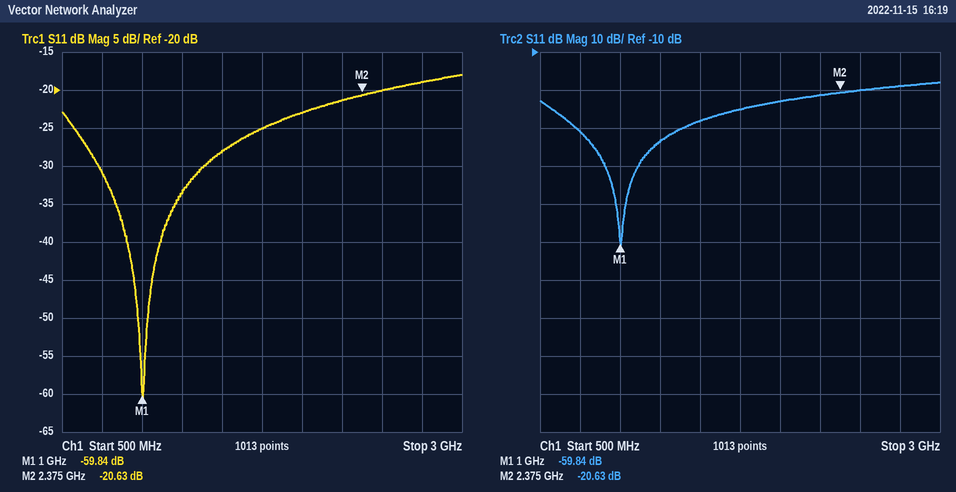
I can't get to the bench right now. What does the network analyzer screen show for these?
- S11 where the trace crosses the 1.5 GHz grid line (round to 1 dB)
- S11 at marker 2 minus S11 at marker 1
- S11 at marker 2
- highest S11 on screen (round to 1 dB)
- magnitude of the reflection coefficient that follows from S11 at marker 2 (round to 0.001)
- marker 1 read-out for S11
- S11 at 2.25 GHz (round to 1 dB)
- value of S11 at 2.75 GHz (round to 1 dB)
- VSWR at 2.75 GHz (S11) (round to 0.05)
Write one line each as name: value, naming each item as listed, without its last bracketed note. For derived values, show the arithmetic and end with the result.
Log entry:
S11 where the trace crosses the 1.5 GHz grid line: -28 dB
S11 at marker 2 minus S11 at marker 1: -20.63 − (-59.84) = 39.21 dB
S11 at marker 2: -20.63 dB
highest S11 on screen: -18 dB
magnitude of the reflection coefficient that follows from S11 at marker 2: 10^(-20.63/20) ≈ 0.093
marker 1 read-out for S11: -59.84 dB
S11 at 2.25 GHz: -21 dB
value of S11 at 2.75 GHz: -19 dB
VSWR at 2.75 GHz (S11): |Γ| = 10^(-19/20) = 0.1122; VSWR = (1 + 0.1122)/(1 − 0.1122) ≈ 1.25
